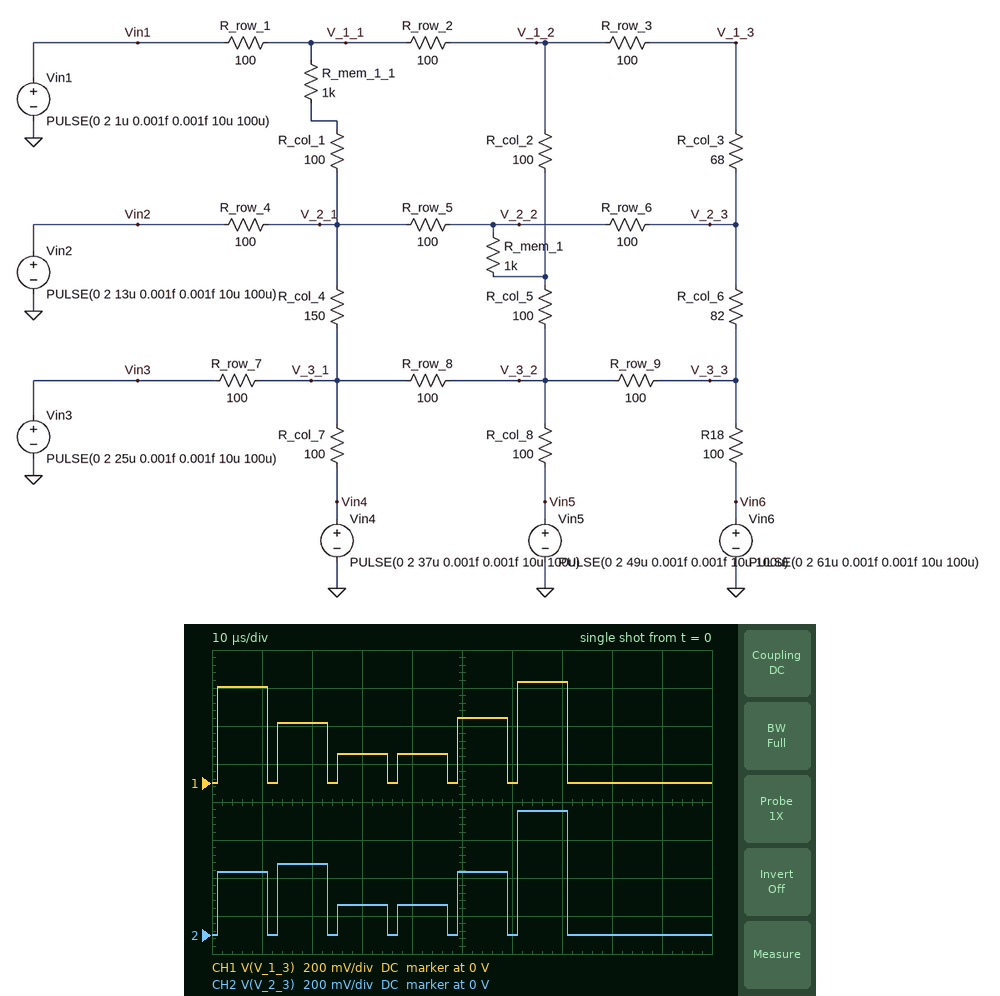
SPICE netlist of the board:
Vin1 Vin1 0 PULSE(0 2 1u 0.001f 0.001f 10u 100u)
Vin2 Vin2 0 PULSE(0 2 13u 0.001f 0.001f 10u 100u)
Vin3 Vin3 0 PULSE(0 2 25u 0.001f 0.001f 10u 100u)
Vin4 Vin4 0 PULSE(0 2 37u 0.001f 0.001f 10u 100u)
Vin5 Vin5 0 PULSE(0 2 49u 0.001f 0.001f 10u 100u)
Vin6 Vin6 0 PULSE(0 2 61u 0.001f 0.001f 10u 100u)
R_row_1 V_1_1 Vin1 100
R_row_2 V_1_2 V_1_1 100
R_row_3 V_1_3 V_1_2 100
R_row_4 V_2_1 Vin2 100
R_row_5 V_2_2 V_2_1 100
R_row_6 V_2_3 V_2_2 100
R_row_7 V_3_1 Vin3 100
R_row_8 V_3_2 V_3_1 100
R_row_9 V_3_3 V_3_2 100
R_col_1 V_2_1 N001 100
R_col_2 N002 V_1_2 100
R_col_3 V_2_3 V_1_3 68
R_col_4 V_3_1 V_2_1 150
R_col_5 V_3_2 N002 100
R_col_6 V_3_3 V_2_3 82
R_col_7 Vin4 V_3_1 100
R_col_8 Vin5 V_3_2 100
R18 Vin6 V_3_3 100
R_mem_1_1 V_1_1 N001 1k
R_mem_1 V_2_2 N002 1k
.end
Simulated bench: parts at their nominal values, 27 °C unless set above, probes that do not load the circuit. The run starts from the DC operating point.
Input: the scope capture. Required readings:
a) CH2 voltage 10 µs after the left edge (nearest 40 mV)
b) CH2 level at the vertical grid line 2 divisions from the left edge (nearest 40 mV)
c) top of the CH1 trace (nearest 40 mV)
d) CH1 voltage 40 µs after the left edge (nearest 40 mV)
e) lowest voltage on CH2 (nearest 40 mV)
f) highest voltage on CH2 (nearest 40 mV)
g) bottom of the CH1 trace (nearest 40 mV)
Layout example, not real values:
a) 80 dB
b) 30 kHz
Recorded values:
a) 320 mV
b) 360 mV
c) 520 mV
d) 160 mV
e) 0 V
f) 640 mV
g) 0 V
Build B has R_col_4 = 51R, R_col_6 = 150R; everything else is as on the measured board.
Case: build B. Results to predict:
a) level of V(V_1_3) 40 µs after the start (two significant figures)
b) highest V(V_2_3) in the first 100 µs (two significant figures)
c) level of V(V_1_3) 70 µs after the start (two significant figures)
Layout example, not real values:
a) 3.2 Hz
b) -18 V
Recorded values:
a) 190 mV
b) 540 mV
c) 450 mV
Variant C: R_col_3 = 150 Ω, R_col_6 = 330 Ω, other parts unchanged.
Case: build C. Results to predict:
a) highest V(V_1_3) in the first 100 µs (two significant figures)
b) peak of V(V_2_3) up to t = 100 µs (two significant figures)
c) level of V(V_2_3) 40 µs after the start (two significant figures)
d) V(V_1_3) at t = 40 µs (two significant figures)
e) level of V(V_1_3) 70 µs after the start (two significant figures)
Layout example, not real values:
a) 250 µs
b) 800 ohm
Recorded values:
a) 660 mV
b) 540 mV
c) 180 mV
d) 160 mV
e) 320 mV
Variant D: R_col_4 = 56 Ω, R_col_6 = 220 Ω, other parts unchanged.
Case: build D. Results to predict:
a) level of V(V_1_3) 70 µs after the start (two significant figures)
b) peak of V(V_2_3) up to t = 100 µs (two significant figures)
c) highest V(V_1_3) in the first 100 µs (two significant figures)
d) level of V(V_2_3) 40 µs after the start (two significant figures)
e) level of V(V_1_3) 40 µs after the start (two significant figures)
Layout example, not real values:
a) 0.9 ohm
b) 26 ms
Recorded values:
a) 400 mV
b) 470 mV
c) 560 mV
d) 210 mV
e) 190 mV
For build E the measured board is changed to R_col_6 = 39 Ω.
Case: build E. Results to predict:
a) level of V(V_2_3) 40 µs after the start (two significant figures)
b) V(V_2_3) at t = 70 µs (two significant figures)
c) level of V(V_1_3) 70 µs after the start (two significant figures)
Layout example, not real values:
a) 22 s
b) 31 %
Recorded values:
a) 150 mV
b) 750 mV
c) 610 mV
